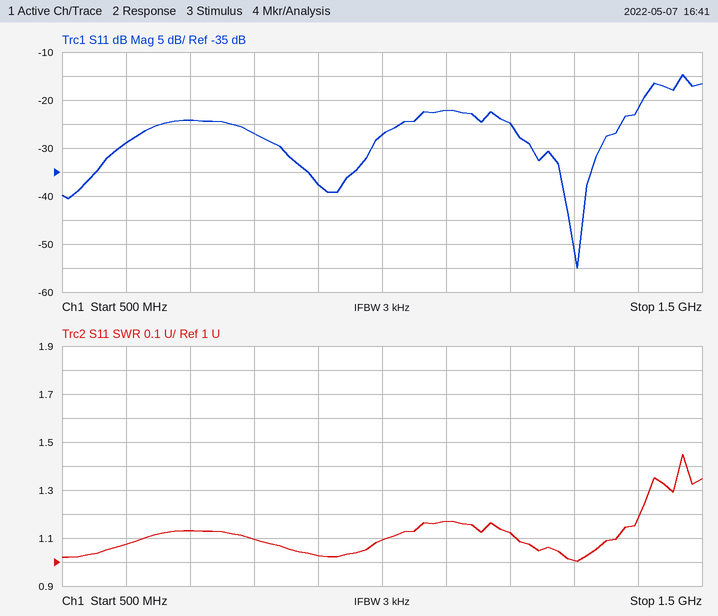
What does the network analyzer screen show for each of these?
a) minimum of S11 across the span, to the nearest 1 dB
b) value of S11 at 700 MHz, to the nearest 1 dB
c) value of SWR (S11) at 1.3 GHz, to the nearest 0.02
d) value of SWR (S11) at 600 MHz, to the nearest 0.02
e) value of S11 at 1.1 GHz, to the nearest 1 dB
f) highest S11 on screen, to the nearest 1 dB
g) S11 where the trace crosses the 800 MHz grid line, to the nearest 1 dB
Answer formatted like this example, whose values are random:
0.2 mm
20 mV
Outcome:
-55 dB
-24 dB
1.00
1.08
-22 dB
-15 dB
-27 dB
